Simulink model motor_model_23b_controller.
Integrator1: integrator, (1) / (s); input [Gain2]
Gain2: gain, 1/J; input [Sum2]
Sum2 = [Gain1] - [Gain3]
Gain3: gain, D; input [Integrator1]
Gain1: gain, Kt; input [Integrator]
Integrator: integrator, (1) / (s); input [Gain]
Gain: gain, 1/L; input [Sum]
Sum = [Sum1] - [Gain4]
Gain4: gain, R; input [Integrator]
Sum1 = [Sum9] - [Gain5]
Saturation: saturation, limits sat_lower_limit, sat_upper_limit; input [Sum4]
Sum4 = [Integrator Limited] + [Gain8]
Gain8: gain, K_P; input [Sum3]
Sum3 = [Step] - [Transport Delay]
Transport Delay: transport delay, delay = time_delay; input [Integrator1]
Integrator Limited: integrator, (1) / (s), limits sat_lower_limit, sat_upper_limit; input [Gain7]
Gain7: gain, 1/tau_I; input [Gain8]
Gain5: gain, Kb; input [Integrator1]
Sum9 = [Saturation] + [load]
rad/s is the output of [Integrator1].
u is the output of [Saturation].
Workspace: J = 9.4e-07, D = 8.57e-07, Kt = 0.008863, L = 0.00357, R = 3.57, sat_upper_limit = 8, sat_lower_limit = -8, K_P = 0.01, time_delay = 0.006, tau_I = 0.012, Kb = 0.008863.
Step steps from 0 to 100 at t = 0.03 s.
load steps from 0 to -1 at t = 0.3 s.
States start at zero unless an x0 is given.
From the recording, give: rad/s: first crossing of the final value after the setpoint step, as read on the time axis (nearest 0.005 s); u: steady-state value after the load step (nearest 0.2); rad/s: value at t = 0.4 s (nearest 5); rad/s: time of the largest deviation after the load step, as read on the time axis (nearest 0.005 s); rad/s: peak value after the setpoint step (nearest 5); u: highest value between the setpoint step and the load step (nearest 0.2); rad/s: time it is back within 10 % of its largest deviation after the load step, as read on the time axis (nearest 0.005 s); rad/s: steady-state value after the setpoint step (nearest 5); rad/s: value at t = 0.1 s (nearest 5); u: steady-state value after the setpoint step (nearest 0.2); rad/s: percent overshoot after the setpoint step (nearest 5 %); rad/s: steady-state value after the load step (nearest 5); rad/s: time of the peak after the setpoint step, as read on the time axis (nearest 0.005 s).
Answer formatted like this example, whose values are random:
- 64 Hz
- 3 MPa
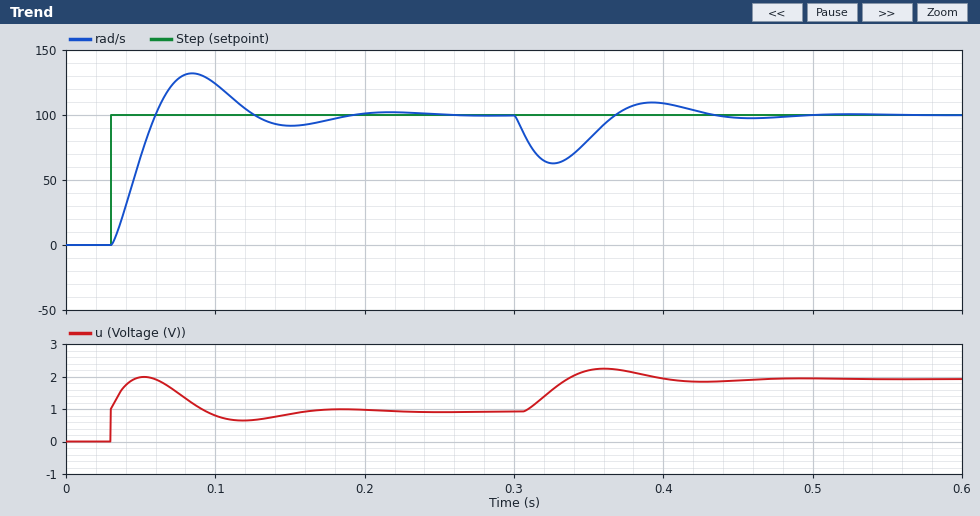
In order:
- 0.060 s
- 2.0
- 110
- 0.325 s
- 130
- 2.0
- 0.420 s
- 100
- 125
- 1.0
- 30 %
- 100
- 0.085 s
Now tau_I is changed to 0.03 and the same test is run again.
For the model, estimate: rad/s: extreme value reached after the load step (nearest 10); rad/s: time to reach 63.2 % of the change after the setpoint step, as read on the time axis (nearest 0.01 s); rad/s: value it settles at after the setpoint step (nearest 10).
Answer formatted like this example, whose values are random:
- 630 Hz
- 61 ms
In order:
- 60
- 0.06 s
- 100
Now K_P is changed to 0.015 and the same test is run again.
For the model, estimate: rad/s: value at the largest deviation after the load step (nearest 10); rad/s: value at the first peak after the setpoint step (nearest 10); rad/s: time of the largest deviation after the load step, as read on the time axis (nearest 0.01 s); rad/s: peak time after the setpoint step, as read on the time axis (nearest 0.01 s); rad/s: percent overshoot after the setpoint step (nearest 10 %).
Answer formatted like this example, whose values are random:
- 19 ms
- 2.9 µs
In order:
- 70
- 140
- 0.32 s
- 0.07 s
- 40 %
